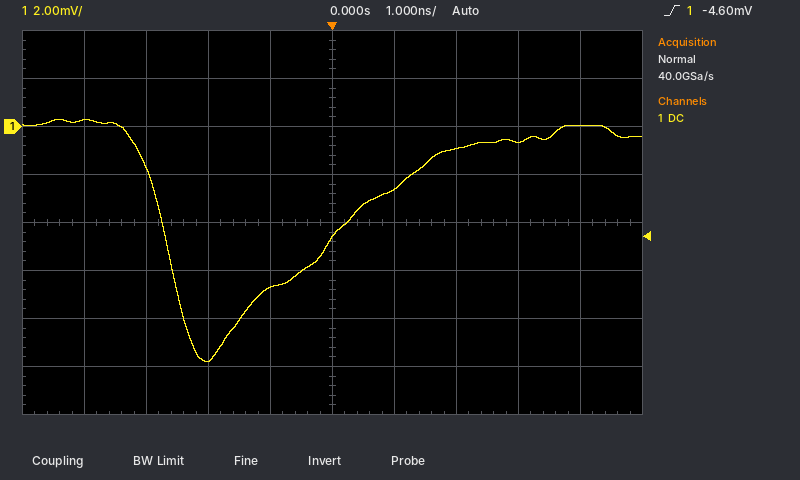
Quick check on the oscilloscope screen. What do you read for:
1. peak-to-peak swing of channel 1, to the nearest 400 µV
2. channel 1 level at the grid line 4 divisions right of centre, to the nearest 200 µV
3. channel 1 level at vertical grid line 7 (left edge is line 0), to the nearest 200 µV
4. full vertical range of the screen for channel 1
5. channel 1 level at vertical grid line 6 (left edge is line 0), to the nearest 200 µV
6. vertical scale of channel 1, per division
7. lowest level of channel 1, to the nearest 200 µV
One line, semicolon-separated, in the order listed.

10.0 mV; 0.0 mV; -1.0 mV; 16 mV; -2.6 mV; 2 mV; -9.8 mV
